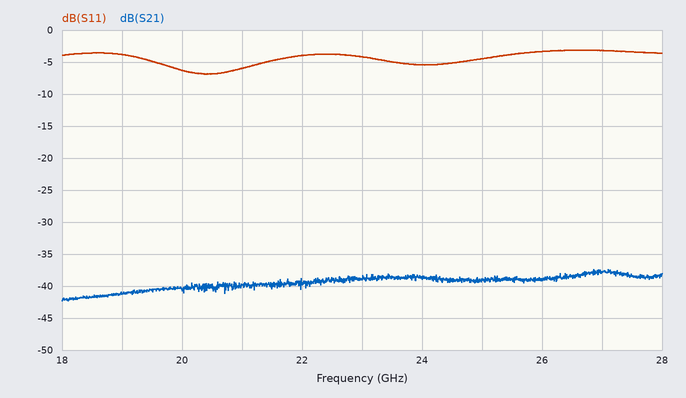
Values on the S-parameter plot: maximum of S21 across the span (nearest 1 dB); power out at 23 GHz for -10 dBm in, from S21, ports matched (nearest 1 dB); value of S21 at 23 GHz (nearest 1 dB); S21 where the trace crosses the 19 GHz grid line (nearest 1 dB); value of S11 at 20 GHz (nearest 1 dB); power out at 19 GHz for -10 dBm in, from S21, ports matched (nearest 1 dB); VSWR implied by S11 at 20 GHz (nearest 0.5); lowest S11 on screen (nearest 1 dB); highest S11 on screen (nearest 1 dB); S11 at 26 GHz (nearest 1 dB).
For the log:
-37 dB
-49 dBm
-39 dB
-41 dB
-6 dB
-51 dBm
3.0
-7 dB
-3 dB
-3 dB
